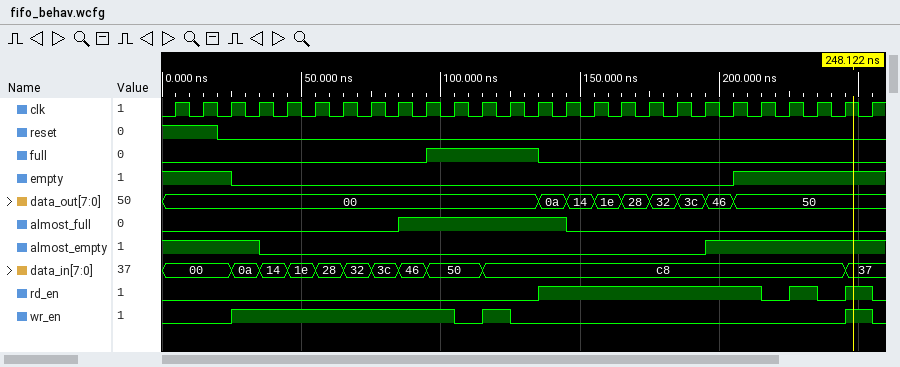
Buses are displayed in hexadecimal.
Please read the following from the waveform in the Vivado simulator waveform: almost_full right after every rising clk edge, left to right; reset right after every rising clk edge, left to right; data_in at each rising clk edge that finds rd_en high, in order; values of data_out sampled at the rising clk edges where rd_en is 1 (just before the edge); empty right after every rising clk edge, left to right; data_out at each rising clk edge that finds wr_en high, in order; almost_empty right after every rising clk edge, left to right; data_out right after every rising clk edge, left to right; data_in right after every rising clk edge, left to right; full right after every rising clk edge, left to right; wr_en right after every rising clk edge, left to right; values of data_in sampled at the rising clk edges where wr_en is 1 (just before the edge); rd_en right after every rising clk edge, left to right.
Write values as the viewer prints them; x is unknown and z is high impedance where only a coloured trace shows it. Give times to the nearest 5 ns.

0 0 0 0 0 0 0 0 1 1 1 1 1 1 0 0 0 0 0 0 0 0 0 0 0 0
1 1 0 0 0 0 0 0 0 0 0 0 0 0 0 0 0 0 0 0 0 0 0 0 0 0
c8, c8, c8, c8, c8, c8, c8, c8, c8, 37
0a, 14, 1e, 28, 32, 3c, 46, 50, 50, 50
1 1 0 0 0 0 0 0 0 0 0 0 0 0 0 0 0 0 0 0 1 1 1 1 1 1
00, 00, 00, 00, 00, 00, 00, 00, 00, 50
1 1 1 0 0 0 0 0 0 0 0 0 0 0 0 0 0 0 0 1 1 1 1 1 1 1
00, 00, 00, 00, 00, 00, 00, 00, 00, 00, 00, 00, 00, 0a, 14, 1e, 28, 32, 3c, 46, 50, 50, 50, 50, 50, 50
00, 00, 0a, 14, 1e, 28, 32, 3c, 46, 50, 50, c8, c8, c8, c8, c8, c8, c8, c8, c8, c8, c8, c8, c8, 37, 37
0 0 0 0 0 0 0 0 0 1 1 1 1 0 0 0 0 0 0 0 0 0 0 0 0 0
0 0 1 1 1 1 1 1 1 1 0 1 0 0 0 0 0 0 0 0 0 0 0 0 1 0
0a, 14, 1e, 28, 32, 3c, 46, 50, c8, 37
0 0 0 0 0 0 0 0 0 0 0 0 0 1 1 1 1 1 1 1 1 0 1 0 1 0
